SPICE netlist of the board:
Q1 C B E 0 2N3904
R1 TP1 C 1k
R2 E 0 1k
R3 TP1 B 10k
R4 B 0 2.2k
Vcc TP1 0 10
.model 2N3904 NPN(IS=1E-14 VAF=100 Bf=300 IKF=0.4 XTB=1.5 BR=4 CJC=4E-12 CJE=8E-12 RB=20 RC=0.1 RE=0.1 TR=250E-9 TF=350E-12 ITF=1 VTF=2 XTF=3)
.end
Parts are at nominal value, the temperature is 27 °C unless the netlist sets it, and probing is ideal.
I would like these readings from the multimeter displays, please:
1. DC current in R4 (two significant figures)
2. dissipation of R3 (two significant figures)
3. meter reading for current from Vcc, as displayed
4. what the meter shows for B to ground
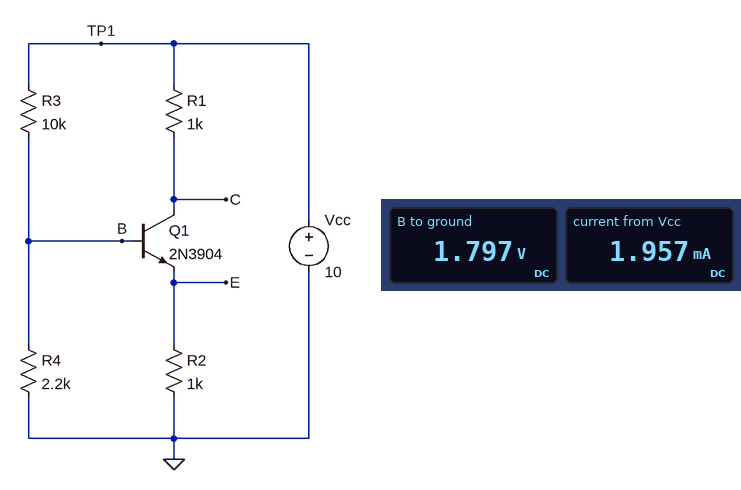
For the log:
820 µA
6.7 mW
1.957 mA
1.797 V
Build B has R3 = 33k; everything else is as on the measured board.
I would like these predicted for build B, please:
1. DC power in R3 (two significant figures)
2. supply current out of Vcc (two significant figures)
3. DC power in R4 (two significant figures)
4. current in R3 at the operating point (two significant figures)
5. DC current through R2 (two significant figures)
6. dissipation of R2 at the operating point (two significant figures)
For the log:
2.7 mW
330 µA
180 µW
280 µA
50 µA
2.5 µW
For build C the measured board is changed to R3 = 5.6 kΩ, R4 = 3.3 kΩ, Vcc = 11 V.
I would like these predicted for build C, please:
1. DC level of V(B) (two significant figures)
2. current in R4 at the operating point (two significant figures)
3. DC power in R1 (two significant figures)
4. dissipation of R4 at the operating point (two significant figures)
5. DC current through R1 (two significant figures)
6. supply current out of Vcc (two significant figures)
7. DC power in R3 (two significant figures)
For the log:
4.1 V
1.2 mA
11 mW
5.0 mW
3.4 mA
4.6 mA
8.6 mW
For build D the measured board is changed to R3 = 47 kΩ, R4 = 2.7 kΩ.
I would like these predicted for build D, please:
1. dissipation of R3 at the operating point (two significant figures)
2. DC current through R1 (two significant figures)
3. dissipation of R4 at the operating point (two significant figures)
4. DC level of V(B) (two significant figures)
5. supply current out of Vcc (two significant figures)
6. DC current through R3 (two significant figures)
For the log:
1.9 mW
9.9 µA
110 µW
540 mV
210 µA
200 µA
